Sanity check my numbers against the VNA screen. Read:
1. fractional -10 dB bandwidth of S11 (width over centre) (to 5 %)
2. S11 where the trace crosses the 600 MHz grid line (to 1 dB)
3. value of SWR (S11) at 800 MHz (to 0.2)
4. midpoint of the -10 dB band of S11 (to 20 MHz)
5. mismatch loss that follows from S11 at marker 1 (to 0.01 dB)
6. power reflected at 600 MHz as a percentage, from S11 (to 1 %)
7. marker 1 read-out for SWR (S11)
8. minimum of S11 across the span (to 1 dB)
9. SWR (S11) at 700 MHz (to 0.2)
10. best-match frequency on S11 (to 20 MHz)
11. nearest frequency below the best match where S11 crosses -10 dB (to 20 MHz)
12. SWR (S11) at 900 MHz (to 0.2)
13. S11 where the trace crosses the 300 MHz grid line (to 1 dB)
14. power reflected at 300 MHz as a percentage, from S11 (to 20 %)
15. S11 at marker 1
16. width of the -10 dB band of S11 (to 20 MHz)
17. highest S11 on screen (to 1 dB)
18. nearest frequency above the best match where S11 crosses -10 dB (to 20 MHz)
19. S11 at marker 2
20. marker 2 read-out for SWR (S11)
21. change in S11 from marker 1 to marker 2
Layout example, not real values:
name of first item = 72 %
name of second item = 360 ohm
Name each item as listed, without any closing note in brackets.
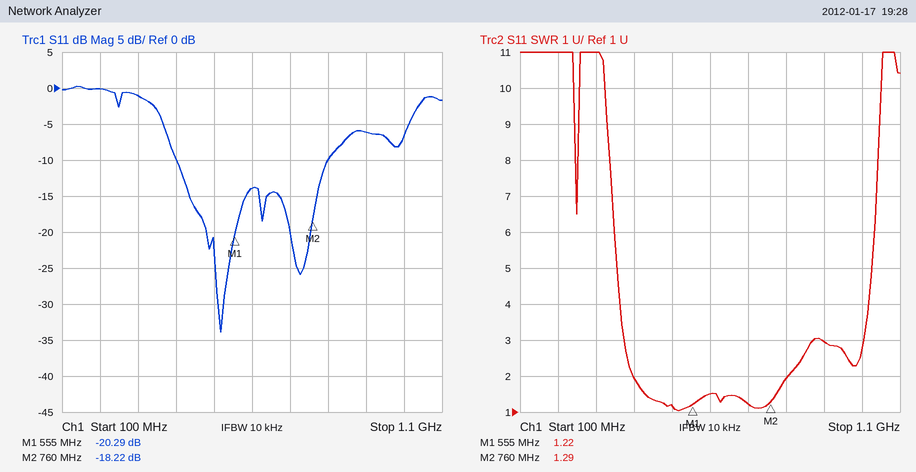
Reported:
fractional -10 dB bandwidth of S11 (width over centre) = 65 %
S11 where the trace crosses the 600 MHz grid line = -14 dB
value of SWR (S11) at 800 MHz = 2.0
midpoint of the -10 dB band of S11 = 600 MHz
mismatch loss that follows from S11 at marker 1 = 0.04 dB
power reflected at 600 MHz as a percentage, from S11 = 4 %
marker 1 read-out for SWR = 1.22
minimum of S11 across the span = -34 dB
SWR (S11) at 700 MHz = 1.2
best-match frequency on S11 = 520 MHz
nearest frequency below the best match where S11 crosses -10 dB = 400 MHz
SWR (S11) at 900 MHz = 3.0
S11 where the trace crosses the 300 MHz grid line = -1 dB
power reflected at 300 MHz as a percentage, from S11 = 80 %
S11 at marker 1 = -20.29 dB
width of the -10 dB band of S11 = 400 MHz
highest S11 on screen = 0 dB
nearest frequency above the best match where S11 crosses -10 dB = 800 MHz
S11 at marker 2 = -18.22 dB
marker 2 read-out for SWR = 1.29
change in S11 from marker 1 to marker 2 = 2.07 dB
